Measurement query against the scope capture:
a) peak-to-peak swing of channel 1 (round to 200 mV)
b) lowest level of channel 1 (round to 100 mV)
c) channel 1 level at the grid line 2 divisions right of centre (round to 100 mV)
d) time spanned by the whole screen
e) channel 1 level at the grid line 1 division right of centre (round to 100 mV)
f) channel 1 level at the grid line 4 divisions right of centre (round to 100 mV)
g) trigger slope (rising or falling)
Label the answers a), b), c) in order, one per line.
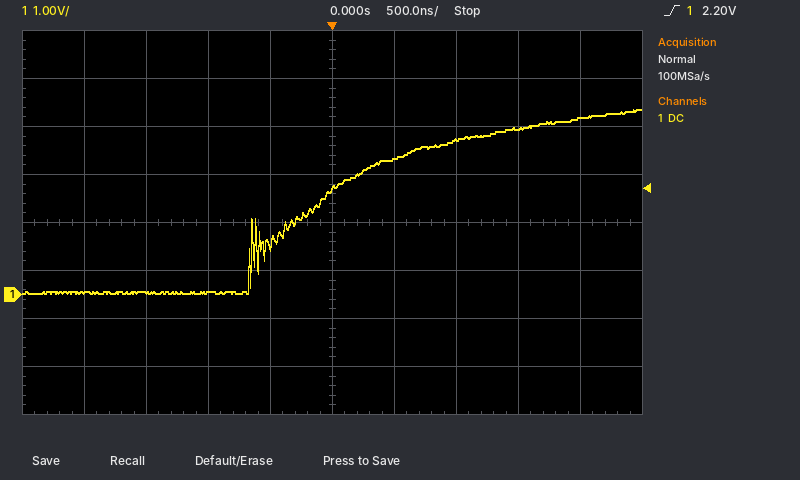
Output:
a) 3.8 V
b) 0.0 V
c) 3.2 V
d) 5 µs
e) 2.8 V
f) 3.7 V
g) rising
